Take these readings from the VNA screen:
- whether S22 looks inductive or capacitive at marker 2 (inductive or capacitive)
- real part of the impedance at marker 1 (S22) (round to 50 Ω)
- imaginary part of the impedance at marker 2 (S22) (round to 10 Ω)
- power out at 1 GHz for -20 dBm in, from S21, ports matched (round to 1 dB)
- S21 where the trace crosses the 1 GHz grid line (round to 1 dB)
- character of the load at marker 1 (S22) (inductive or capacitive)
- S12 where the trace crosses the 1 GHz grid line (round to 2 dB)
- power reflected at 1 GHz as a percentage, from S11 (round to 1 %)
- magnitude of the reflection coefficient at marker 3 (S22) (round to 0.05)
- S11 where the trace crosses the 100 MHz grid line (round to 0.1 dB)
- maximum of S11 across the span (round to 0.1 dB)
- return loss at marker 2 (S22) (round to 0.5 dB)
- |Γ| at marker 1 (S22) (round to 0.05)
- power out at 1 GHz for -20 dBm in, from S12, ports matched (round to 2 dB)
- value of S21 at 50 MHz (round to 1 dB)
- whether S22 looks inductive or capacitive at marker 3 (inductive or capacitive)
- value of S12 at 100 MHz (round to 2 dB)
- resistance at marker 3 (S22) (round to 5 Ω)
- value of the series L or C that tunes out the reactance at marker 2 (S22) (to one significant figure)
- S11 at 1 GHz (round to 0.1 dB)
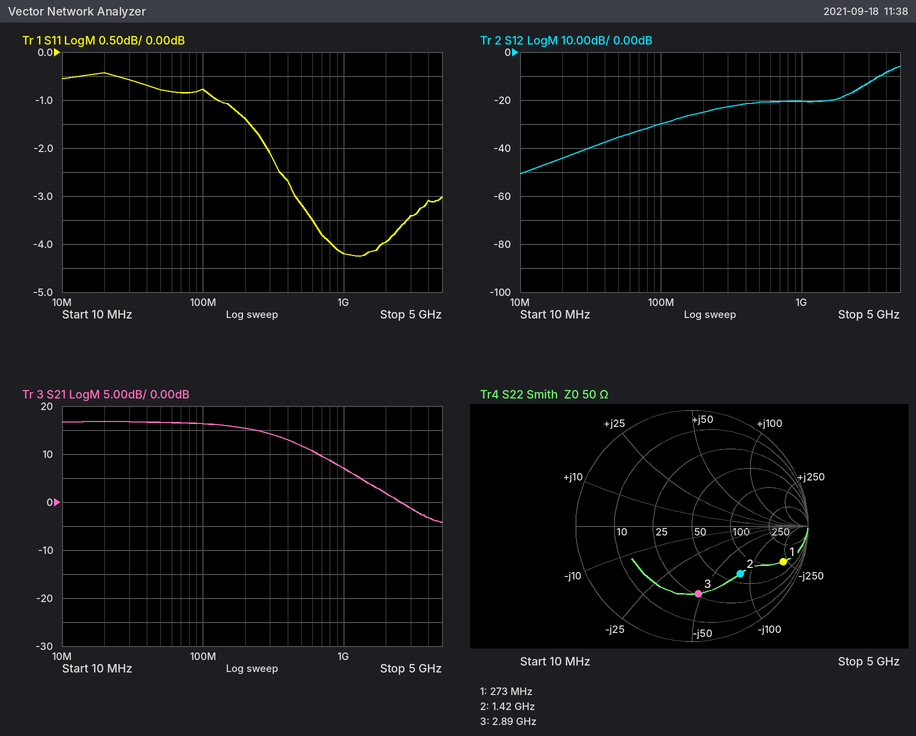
capacitive
100 Ω
-80 Ω
-13 dBm
7 dB
capacitive
-20 dB
38 %
0.60
-0.8 dB
-0.4 dB
4.5 dB
0.85
-40 dBm
17 dB
capacitive
-30 dB
25 Ω
9 nH
-4.2 dB
